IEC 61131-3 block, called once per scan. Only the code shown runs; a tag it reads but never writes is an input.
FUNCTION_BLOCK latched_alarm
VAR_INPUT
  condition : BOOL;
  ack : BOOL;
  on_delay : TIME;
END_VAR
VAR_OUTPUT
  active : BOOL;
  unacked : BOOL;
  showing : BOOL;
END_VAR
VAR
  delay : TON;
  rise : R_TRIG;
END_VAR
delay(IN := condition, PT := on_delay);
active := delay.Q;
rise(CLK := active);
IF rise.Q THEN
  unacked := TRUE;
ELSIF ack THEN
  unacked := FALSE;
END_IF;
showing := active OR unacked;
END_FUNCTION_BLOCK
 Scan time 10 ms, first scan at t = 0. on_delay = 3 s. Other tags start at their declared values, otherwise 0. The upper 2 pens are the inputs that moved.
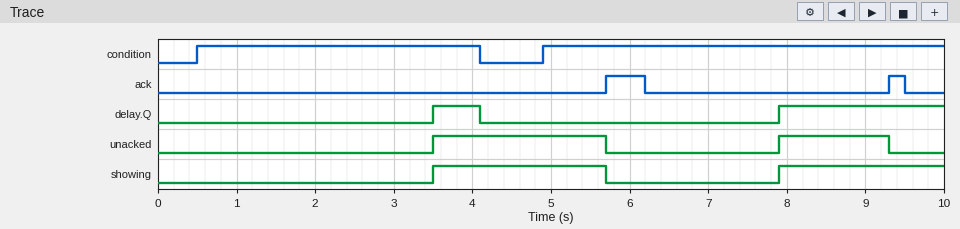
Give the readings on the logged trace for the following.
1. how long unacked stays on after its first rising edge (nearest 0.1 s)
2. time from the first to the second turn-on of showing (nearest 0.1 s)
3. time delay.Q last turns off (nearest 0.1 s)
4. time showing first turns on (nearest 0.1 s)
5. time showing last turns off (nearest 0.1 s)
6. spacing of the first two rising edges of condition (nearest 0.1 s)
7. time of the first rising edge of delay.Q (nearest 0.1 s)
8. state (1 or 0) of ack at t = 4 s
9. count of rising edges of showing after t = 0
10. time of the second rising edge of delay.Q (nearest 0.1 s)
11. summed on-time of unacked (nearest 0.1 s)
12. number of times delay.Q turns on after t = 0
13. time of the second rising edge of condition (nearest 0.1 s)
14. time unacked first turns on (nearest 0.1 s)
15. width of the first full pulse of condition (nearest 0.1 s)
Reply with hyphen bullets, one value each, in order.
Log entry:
- 2.2 s
- 4.4 s
- 4.1 s
- 3.5 s
- 5.7 s
- 4.4 s
- 3.5 s
- 0
- 2
- 7.9 s
- 3.6 s
- 2
- 4.9 s
- 3.5 s
- 3.6 s
